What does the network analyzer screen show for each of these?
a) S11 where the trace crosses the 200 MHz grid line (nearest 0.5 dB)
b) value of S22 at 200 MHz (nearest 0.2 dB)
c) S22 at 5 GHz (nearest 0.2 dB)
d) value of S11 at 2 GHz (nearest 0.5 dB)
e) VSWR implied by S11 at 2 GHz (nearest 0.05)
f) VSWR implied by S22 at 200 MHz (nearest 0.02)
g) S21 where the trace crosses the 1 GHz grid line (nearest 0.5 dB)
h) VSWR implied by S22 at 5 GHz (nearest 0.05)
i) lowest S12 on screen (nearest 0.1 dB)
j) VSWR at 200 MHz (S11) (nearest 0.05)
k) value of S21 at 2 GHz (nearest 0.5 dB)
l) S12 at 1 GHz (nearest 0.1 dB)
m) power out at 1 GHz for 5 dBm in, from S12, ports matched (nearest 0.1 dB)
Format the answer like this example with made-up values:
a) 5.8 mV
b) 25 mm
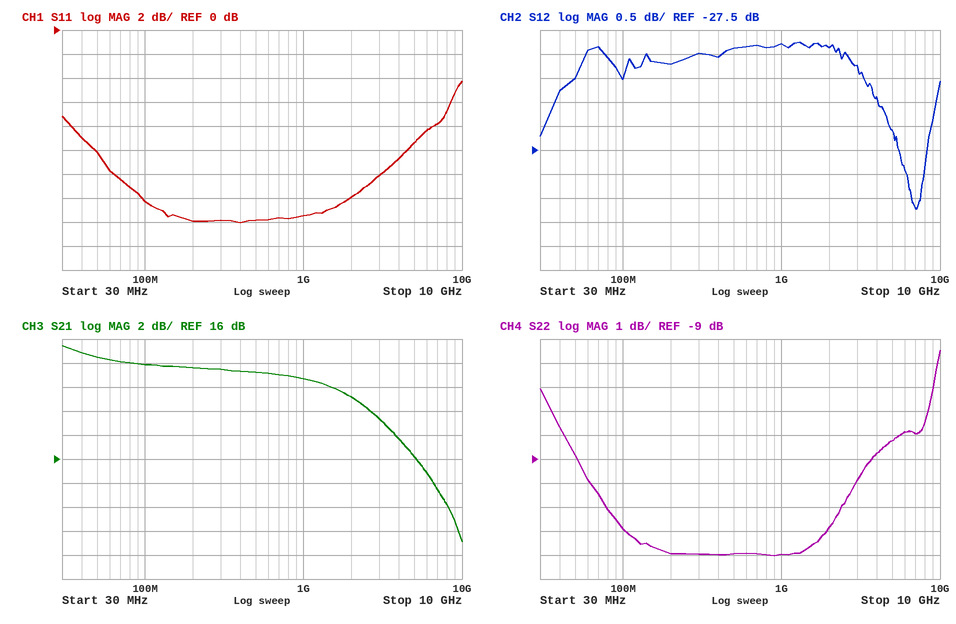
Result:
a) -16.0 dB
b) -13.0 dB
c) -8.2 dB
d) -14.0 dB
e) 1.50
f) 1.58
g) 22.5 dB
h) 2.25
i) -28.7 dB
j) 1.40
k) 21.0 dB
l) -25.3 dB
m) -20.3 dBm
